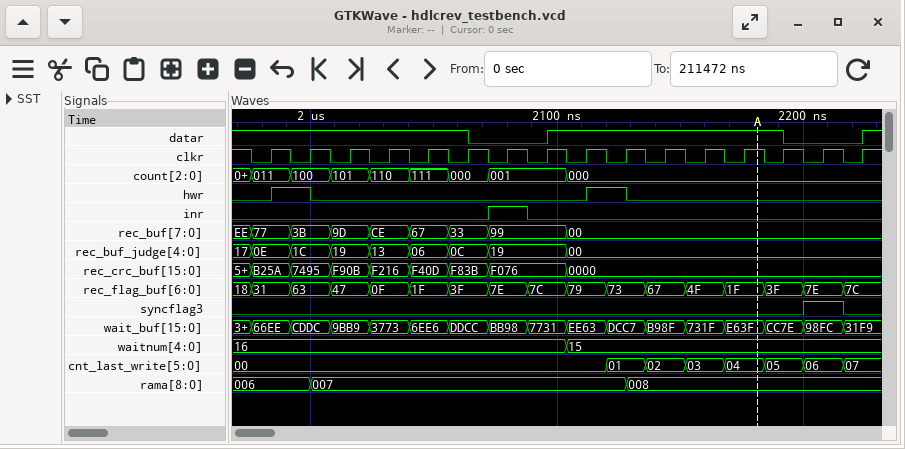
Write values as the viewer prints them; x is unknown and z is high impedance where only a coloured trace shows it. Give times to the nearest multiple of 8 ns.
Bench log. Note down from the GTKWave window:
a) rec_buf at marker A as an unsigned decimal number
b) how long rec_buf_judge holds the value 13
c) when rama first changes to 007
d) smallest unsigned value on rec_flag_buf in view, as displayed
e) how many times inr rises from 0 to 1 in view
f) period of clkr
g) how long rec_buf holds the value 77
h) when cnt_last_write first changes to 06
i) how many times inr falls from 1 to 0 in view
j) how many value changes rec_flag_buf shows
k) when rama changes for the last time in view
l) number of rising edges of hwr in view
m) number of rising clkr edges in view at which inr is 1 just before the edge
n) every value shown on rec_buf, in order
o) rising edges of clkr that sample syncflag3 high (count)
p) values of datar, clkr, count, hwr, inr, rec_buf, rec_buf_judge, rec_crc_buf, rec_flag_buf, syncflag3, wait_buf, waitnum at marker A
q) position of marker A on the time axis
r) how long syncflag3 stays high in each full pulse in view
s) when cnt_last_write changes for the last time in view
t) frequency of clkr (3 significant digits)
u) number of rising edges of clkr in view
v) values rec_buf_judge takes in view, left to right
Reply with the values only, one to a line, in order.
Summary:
0
16 ns
2000 ns
0F
1
16 ns
16 ns
2200 ns
1
16
2128 ns
2
1
EE, 77, 3B, 9D, CE, 67, 33, 99, 00
1
datar=1, clkr=1, count=000, hwr=0, inr=0, rec_buf=00, rec_buf_judge=00, rec_crc_buf=0000, rec_flag_buf=1F, syncflag3=0, wait_buf=E63F, waitnum=15
2184 ns
16 ns
2216 ns
62.5 MHz
16
17, 0E, 1C, 19, 13, 06, 0C, 19, 00
